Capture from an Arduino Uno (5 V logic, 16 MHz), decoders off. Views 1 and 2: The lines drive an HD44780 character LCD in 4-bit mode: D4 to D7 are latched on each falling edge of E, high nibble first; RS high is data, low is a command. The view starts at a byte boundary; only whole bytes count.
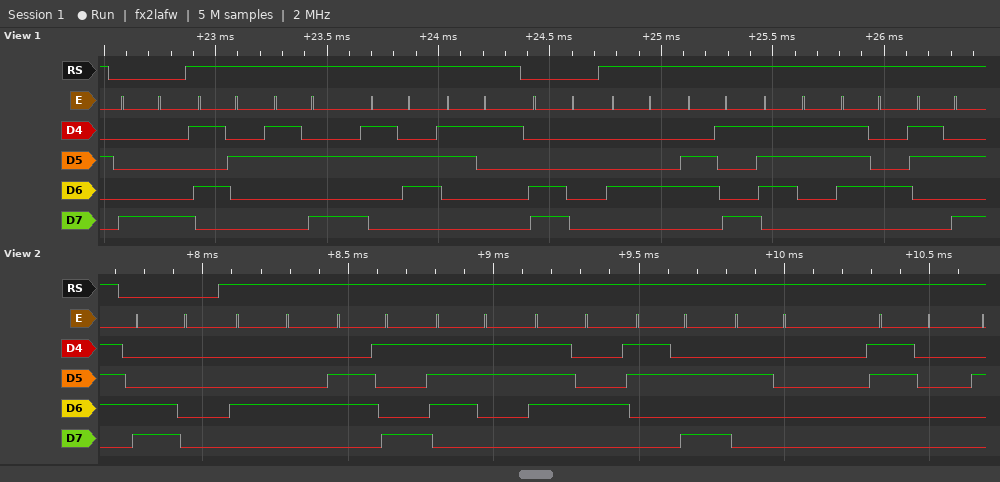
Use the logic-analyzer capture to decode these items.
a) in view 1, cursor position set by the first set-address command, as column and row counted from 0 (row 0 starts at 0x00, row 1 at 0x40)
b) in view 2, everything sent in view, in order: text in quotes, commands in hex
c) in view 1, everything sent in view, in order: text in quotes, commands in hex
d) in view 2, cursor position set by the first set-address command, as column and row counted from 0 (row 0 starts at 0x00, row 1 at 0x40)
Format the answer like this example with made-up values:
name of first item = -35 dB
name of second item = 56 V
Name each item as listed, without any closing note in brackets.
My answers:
in view 1, cursor position set by the first set-address command, as column and row counted from 0 = column 8, row 0
in view 2, everything sent in view, in order: text in quotes, commands in hex = 0xC0 "Dist: 0"
in view 1, everything sent in view, in order: text in quotes, commands in hex = 0x88 "R:61" 0xC0 "Dist:"
in view 2, cursor position set by the first set-address command, as column and row counted from 0 = column 0, row 1
